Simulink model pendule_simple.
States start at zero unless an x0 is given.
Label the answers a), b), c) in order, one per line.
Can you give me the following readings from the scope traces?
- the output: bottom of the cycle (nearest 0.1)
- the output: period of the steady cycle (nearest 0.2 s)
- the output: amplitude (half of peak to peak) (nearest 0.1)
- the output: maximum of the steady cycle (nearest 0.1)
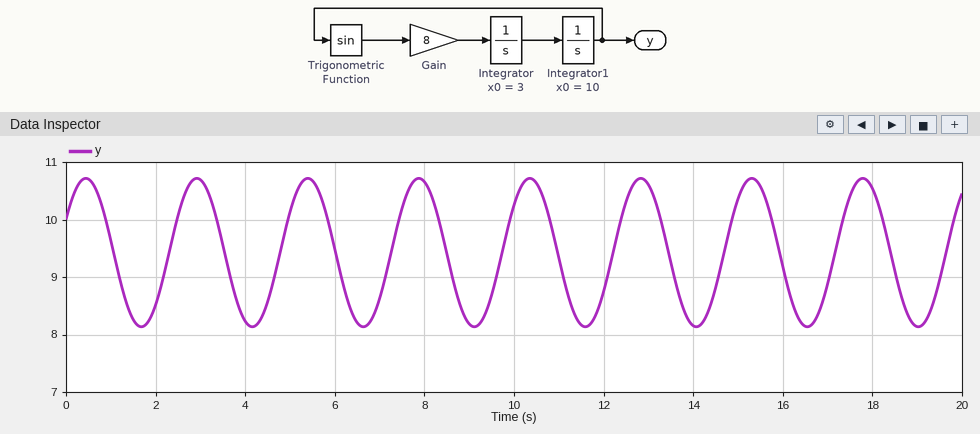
a) 8.1
b) 2.4 s
c) 1.3
d) 10.7
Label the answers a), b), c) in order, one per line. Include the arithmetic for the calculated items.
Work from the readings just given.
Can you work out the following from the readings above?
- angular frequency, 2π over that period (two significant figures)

a) 2π / 2.4 = 2.6 rad/s
